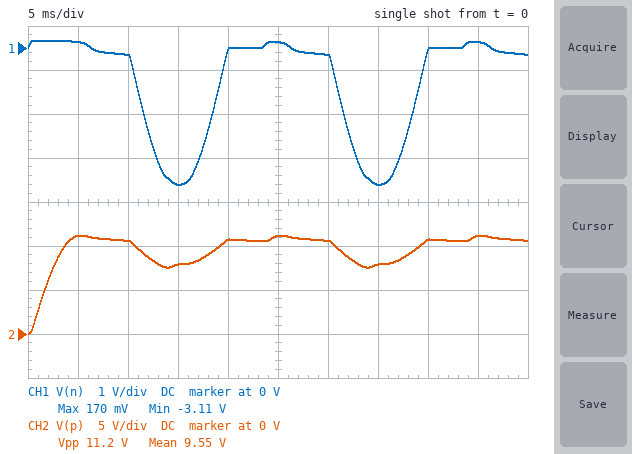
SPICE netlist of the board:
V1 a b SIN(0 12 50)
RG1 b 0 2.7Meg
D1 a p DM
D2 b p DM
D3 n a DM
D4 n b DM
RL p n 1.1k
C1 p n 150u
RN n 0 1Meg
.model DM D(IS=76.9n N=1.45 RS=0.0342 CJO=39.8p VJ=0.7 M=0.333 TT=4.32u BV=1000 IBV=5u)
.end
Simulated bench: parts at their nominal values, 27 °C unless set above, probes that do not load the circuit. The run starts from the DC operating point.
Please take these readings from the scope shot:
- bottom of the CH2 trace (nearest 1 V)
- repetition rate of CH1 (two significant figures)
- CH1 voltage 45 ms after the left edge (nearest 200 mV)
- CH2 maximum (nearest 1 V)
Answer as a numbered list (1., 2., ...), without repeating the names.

1. 0 V
2. 50 Hz
3. 200 mV
4. 11 V
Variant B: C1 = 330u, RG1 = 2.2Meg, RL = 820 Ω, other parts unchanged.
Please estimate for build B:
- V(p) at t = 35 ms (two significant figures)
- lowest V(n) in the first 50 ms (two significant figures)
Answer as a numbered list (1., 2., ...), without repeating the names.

1. 7.4 V
2. -3.6 V
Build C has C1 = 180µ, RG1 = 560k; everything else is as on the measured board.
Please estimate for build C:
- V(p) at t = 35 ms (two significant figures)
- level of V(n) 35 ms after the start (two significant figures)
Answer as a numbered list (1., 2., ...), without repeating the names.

1. 3.6 V
2. -7.4 V
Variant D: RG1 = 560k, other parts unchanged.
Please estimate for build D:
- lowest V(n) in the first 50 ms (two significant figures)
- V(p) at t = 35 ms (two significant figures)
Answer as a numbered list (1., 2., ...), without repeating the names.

1. -7.4 V
2. 3.6 V
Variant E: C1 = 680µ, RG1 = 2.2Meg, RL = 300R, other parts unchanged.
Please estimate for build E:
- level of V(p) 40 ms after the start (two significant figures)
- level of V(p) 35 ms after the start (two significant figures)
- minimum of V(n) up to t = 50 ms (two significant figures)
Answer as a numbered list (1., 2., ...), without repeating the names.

1. 11 V
2. 7.3 V
3. -3.6 V
